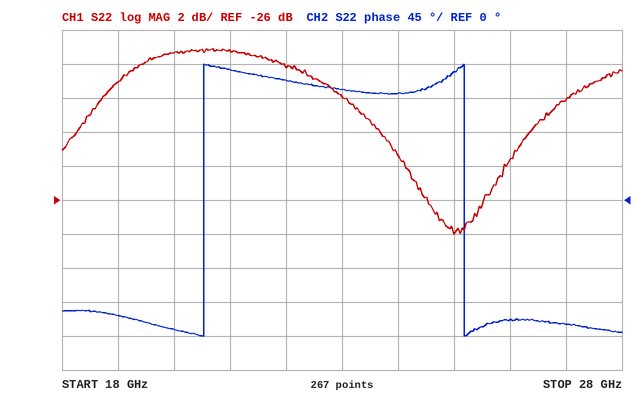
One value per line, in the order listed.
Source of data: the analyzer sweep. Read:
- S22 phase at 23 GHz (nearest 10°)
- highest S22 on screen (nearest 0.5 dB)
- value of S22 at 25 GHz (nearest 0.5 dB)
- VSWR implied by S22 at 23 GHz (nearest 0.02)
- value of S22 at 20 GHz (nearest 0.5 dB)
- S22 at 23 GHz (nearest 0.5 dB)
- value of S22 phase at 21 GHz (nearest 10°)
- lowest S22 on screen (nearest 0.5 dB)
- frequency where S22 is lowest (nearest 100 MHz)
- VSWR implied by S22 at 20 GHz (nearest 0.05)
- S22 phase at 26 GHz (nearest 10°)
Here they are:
150°
-17.0 dB
-28.0 dB
1.22
-17.5 dB
-20.0 dB
170°
-28.0 dB
25.0 GHz
1.30
-160°
